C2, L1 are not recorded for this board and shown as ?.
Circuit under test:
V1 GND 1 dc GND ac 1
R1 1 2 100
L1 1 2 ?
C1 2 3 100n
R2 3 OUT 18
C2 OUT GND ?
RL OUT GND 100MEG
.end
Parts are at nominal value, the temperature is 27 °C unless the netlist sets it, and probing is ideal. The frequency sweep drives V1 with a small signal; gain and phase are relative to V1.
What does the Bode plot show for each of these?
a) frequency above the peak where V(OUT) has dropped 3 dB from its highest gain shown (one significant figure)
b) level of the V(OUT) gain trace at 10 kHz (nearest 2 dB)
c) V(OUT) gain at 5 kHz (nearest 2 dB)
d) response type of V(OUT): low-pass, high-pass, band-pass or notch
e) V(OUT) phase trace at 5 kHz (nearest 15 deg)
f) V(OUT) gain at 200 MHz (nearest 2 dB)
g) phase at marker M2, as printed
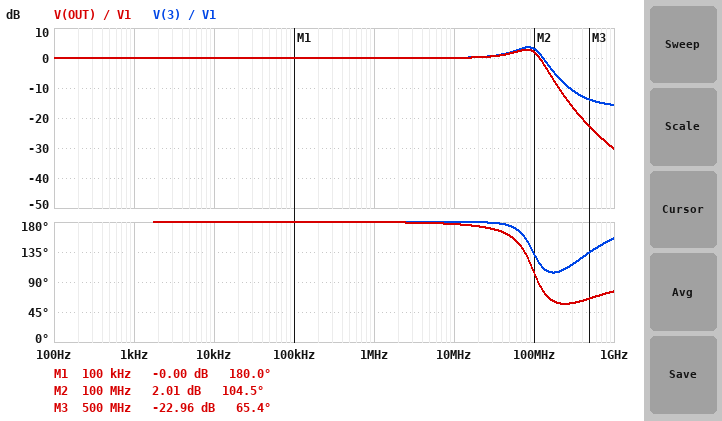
100 MHz
0 dB
0 dB
low-pass
180 deg
-10 dB
104.5 deg
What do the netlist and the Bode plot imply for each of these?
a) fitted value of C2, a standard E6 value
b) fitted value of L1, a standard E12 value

47 pF
47 nH
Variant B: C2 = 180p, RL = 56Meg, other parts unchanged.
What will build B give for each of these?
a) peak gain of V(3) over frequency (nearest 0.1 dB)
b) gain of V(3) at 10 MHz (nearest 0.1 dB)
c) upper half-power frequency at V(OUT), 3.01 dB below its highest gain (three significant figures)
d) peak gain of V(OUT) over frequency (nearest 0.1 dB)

2.2 dB
0.3 dB
57.1 MHz
0.5 dB
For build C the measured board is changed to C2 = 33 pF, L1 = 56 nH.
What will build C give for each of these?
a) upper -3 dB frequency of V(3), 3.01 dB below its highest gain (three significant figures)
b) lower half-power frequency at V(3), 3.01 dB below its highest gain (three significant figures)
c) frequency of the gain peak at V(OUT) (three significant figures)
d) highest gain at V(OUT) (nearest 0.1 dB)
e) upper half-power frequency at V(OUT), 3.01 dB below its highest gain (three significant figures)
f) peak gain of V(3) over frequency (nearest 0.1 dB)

135 MHz
35.0 MHz
92.0 MHz
3.3 dB
131 MHz
3.8 dB
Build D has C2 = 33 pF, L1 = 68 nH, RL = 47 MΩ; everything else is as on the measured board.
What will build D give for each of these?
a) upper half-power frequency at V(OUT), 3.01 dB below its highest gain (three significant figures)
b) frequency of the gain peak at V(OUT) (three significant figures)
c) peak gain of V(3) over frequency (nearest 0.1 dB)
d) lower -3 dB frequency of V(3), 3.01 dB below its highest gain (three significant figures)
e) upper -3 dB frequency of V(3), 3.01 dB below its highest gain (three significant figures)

120 MHz
83.8 MHz
3.8 dB
31.6 MHz
123 MHz
